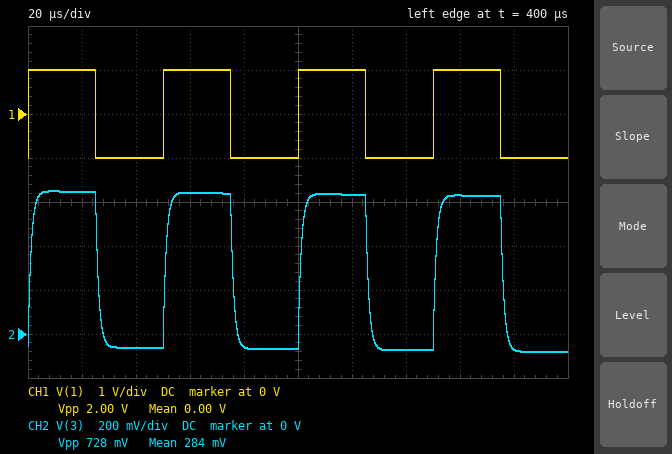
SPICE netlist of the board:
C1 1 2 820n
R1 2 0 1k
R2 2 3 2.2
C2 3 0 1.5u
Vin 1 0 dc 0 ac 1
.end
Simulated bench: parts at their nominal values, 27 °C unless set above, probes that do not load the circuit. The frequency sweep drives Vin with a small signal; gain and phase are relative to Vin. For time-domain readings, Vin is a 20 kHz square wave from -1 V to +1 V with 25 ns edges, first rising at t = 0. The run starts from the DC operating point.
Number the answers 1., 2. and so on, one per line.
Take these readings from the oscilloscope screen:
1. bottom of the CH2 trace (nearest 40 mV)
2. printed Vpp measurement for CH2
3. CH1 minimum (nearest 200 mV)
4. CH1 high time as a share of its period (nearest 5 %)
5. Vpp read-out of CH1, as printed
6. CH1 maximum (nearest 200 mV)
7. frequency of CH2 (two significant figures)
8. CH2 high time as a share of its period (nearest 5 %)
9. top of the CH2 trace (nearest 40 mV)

1. -80 mV
2. 728 mV
3. -1.0 V
4. 50 %
5. 2.00 V
6. 1.0 V
7. 20 kHz
8. 50 %
9. 640 mV
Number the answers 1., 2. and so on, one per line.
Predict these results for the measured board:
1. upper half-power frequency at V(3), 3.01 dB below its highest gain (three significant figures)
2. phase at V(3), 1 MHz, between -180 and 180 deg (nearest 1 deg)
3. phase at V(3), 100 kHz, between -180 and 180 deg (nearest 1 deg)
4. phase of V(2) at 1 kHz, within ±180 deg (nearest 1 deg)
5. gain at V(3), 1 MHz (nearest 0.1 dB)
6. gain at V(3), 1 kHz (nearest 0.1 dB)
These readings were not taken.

1. 137 kHz
2. -82 deg
3. -36 deg
4. 5 deg
5. -26.4 dB
6. -9.1 dB
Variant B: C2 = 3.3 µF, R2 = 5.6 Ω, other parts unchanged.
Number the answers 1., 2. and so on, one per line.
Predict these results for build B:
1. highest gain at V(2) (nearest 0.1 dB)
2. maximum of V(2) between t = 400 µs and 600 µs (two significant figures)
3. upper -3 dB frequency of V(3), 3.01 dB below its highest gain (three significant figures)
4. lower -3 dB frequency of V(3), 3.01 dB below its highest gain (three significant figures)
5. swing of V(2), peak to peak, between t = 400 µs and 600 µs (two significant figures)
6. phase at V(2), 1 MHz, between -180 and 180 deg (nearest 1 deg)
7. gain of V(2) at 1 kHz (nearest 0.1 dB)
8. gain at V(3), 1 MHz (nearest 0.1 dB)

1. 0 dB
2. 2.0 V
3. 43.5 kHz
4. 38.4 Hz
5. 3.6 V
6. 2 deg
7. -14.0 dB
8. -41.3 dB
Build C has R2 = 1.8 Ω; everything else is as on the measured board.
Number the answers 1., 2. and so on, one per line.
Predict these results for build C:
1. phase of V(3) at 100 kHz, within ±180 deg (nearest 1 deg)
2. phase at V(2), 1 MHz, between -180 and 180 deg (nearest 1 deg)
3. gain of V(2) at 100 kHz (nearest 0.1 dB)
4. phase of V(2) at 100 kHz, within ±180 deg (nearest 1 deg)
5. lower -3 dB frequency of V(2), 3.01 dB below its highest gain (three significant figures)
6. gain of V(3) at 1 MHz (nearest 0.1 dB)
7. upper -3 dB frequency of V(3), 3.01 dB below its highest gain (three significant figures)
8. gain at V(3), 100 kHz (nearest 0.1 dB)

1. -31 deg
2. 6 deg
3. -4.5 dB
4. 29 deg
5. 145 kHz
6. -24.7 dB
7. 167 kHz
8. -10.4 dB
